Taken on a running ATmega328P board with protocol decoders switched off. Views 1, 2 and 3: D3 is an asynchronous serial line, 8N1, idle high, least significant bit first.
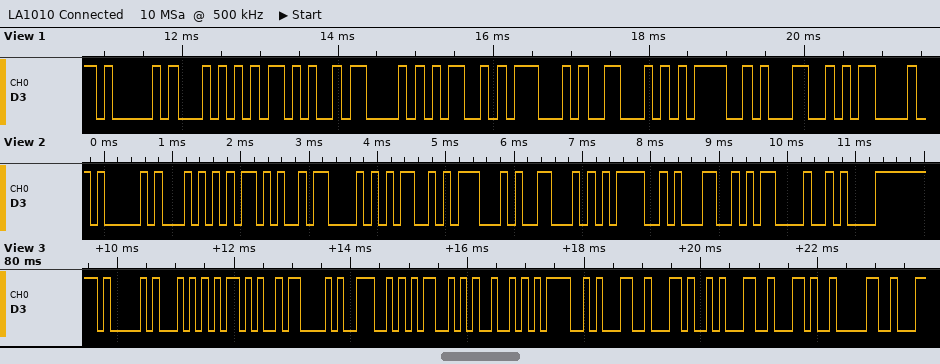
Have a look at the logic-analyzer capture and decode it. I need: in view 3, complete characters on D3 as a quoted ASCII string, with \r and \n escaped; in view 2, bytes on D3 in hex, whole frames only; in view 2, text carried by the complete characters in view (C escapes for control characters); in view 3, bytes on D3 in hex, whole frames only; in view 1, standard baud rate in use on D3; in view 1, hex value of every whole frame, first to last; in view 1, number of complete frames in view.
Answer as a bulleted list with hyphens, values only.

- "AT+CNMI=1,1,0"
- 41 54 2B 43 4D 47 46 3D 31 0D 0A
- "AT+CMGF=1\r\n"
- 0x41 0x54 0x2B 0x43 0x4E 0x4D 0x49 0x3D 0x31 0x2C 0x31 0x2C 0x30
- 9600 baud
- 0x41 0x54 0x2B 0x43 0x4D 0x47 0x46 0x3D 0x31 0x0D
- 10
